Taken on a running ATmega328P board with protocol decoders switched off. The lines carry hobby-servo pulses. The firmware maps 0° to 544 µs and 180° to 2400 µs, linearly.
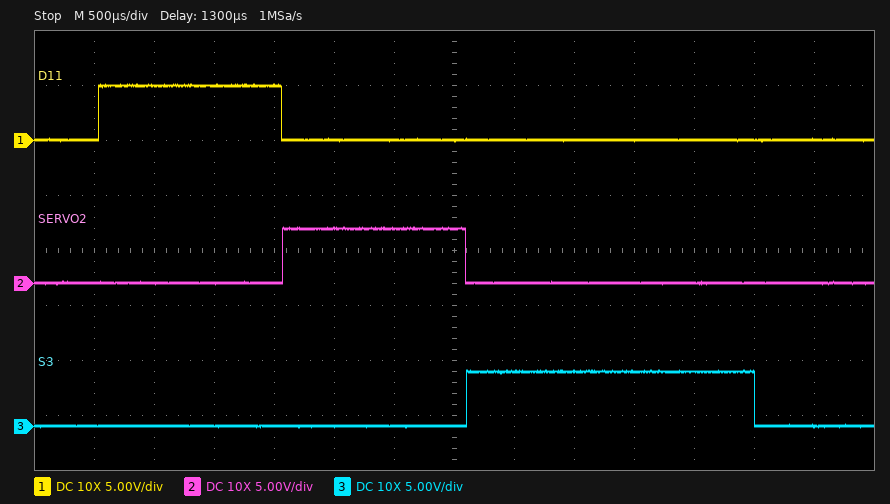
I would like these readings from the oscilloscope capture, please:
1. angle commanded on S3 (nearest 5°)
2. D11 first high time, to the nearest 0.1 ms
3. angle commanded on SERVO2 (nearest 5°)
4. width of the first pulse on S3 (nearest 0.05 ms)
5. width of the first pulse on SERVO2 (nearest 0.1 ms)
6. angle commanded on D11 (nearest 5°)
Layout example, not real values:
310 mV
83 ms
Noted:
180°
1.5 ms
95°
2.40 ms
1.5 ms
95°
